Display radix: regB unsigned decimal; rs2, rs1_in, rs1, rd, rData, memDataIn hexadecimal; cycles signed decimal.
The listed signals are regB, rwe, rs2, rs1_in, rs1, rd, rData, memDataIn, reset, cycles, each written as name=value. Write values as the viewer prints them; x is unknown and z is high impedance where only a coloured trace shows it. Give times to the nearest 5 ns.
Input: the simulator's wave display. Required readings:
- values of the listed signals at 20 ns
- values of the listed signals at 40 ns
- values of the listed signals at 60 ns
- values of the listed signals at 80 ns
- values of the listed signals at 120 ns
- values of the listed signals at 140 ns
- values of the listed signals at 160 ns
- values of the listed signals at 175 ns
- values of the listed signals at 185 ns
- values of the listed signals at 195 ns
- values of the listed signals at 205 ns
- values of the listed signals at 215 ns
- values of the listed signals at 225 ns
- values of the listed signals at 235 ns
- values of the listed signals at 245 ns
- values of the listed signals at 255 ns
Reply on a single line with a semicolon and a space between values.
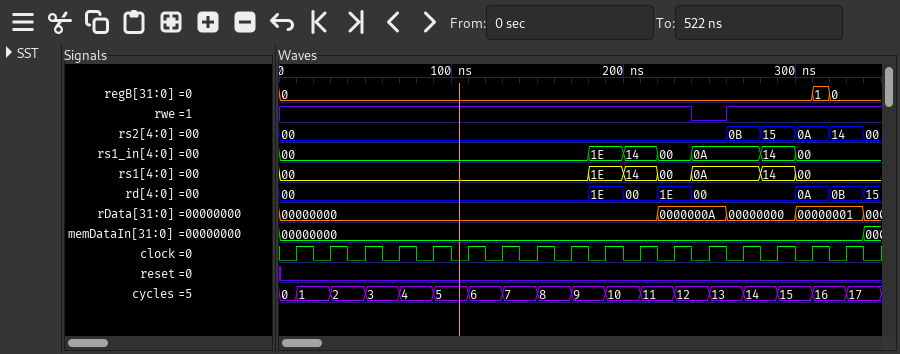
regB=0, rwe=1, rs2=00, rs1_in=00, rs1=00, rd=00, rData=00000000, memDataIn=00000000, reset=0, cycles=1; regB=0, rwe=1, rs2=00, rs1_in=00, rs1=00, rd=00, rData=00000000, memDataIn=00000000, reset=0, cycles=2; regB=0, rwe=1, rs2=00, rs1_in=00, rs1=00, rd=00, rData=00000000, memDataIn=00000000, reset=0, cycles=3; regB=0, rwe=1, rs2=00, rs1_in=00, rs1=00, rd=00, rData=00000000, memDataIn=00000000, reset=0, cycles=4; regB=0, rwe=1, rs2=00, rs1_in=00, rs1=00, rd=00, rData=00000000, memDataIn=00000000, reset=0, cycles=6; regB=0, rwe=1, rs2=00, rs1_in=00, rs1=00, rd=00, rData=00000000, memDataIn=00000000, reset=0, cycles=7; regB=0, rwe=1, rs2=00, rs1_in=00, rs1=00, rd=00, rData=00000000, memDataIn=00000000, reset=0, cycles=8; regB=0, rwe=1, rs2=00, rs1_in=00, rs1=00, rd=00, rData=00000000, memDataIn=00000000, reset=0, cycles=9; regB=0, rwe=1, rs2=00, rs1_in=1E, rs1=1E, rd=1E, rData=00000000, memDataIn=00000000, reset=0, cycles=9; regB=0, rwe=1, rs2=00, rs1_in=1E, rs1=1E, rd=1E, rData=00000000, memDataIn=00000000, reset=0, cycles=10; regB=0, rwe=1, rs2=00, rs1_in=14, rs1=14, rd=00, rData=00000000, memDataIn=00000000, reset=0, cycles=10; regB=0, rwe=1, rs2=00, rs1_in=14, rs1=14, rd=00, rData=00000000, memDataIn=00000000, reset=0, cycles=11; regB=0, rwe=1, rs2=00, rs1_in=00, rs1=00, rd=1E, rData=0000000A, memDataIn=00000000, reset=0, cycles=11; regB=0, rwe=1, rs2=00, rs1_in=00, rs1=00, rd=1E, rData=0000000A, memDataIn=00000000, reset=0, cycles=12; regB=0, rwe=0, rs2=00, rs1_in=0A, rs1=0A, rd=00, rData=0000000A, memDataIn=00000000, reset=0, cycles=12; regB=0, rwe=0, rs2=00, rs1_in=0A, rs1=0A, rd=00, rData=0000000A, memDataIn=00000000, reset=0, cycles=13
